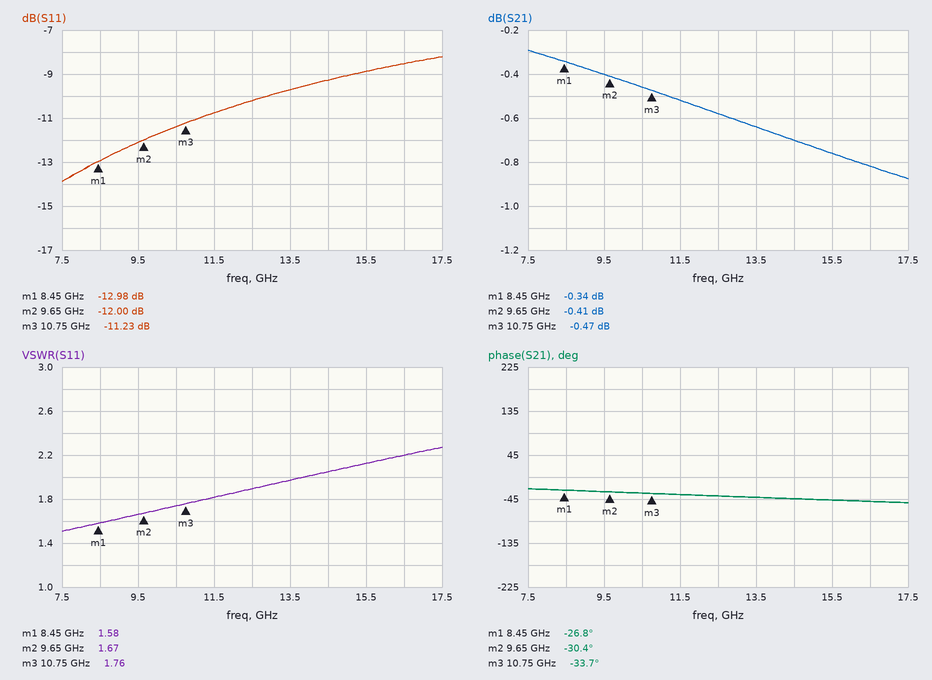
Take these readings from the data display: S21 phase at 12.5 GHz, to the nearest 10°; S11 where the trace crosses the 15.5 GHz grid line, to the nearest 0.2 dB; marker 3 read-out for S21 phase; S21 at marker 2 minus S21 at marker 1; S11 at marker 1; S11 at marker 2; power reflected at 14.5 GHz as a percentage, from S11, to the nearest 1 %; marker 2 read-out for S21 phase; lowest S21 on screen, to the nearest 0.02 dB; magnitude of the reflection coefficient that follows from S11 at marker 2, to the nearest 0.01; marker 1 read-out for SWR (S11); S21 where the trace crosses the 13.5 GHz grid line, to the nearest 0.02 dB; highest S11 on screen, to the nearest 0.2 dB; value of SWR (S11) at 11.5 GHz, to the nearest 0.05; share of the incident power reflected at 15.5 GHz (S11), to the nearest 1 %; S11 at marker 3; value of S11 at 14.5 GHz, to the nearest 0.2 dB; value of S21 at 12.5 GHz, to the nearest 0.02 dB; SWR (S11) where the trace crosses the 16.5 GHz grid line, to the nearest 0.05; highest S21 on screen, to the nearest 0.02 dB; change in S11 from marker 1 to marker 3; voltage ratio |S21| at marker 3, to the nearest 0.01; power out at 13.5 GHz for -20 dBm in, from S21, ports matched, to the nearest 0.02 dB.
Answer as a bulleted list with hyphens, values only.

- -40°
- -8.8 dB
- -33.7°
- -0.07 dB
- -12.98 dB
- -12.00 dB
- 12 %
- -30.4°
- -0.88 dB
- 0.25
- 1.58
- -0.64 dB
- -8.2 dB
- 1.80
- 13 %
- -11.23 dB
- -9.2 dB
- -0.58 dB
- 2.20
- -0.30 dB
- 1.75 dB
- 0.95
- -20.64 dBm
